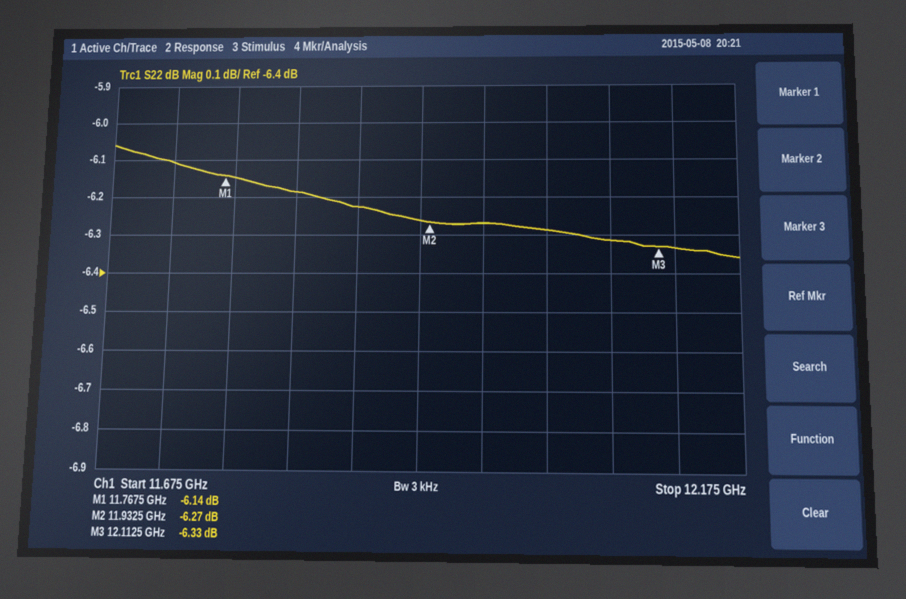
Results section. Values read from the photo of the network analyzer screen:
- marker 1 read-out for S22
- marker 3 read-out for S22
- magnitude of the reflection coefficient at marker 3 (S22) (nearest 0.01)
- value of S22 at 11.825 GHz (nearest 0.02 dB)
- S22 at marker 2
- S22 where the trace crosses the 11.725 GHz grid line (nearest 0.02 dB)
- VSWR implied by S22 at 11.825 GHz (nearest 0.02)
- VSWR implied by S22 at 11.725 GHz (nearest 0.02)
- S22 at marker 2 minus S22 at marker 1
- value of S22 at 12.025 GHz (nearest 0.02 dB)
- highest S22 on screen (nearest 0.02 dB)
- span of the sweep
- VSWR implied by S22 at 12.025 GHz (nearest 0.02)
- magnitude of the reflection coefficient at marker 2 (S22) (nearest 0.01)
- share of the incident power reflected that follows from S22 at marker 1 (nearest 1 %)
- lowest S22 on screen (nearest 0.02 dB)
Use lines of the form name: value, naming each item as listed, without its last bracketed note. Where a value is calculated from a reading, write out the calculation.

marker 1 read-out for S22: -6.14 dB
marker 3 read-out for S22: -6.33 dB
magnitude of the reflection coefficient at marker 3 (S22): 10^(-6.33/20) ≈ 0.48
value of S22 at 11.825 GHz: -6.18 dB
S22 at marker 2: -6.27 dB
S22 where the trace crosses the 11.725 GHz grid line: -6.10 dB
VSWR implied by S22 at 11.825 GHz: |Γ| = 10^(-6.18/20) = 0.4909; VSWR = (1 + 0.4909)/(1 − 0.4909) ≈ 2.93, so 2.92 to the nearest 0.02
VSWR implied by S22 at 11.725 GHz: |Γ| = 10^(-6.1/20) = 0.4955; VSWR = (1 + 0.4955)/(1 − 0.4955) ≈ 2.96
S22 at marker 2 minus S22 at marker 1: -6.27 − (-6.14) = -0.13 dB
value of S22 at 12.025 GHz: -6.28 dB
highest S22 on screen: -6.06 dB
span of the sweep: 500 MHz
VSWR implied by S22 at 12.025 GHz: |Γ| = 10^(-6.28/20) = 0.4853; VSWR = (1 + 0.4853)/(1 − 0.4853) ≈ 2.89, so 2.88 to the nearest 0.02
magnitude of the reflection coefficient at marker 2 (S22): 10^(-6.27/20) ≈ 0.49
share of the incident power reflected that follows from S22 at marker 1: 10^(-6.14/10) ≈ 24 %
lowest S22 on screen: -6.36 dB
